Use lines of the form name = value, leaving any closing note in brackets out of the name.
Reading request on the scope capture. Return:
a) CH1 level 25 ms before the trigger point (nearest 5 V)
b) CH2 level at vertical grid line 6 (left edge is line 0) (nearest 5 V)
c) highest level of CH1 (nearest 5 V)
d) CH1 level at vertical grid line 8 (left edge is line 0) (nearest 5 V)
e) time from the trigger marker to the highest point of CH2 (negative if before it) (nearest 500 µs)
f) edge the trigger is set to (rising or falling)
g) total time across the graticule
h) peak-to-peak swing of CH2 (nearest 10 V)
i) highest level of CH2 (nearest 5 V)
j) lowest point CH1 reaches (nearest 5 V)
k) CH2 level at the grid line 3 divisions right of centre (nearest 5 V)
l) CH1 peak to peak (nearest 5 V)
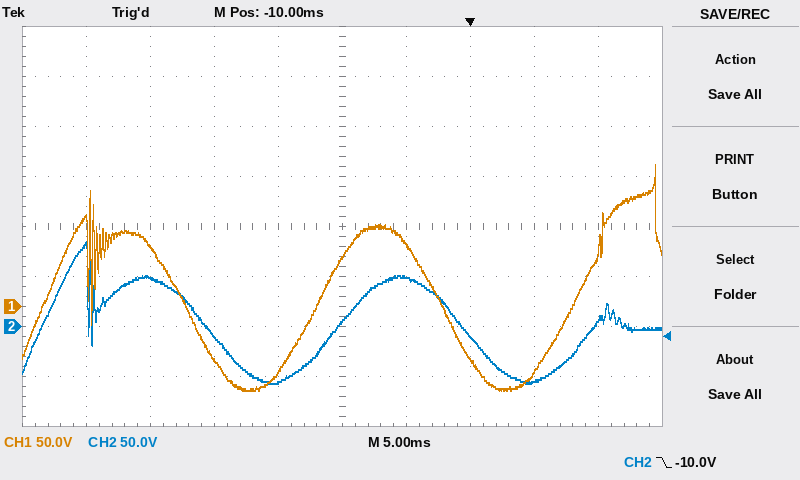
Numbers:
CH1 level 25 ms before the trigger point = 60 V
CH2 level at vertical grid line 6 (left edge is line 0) = 50 V
highest level of CH1 = 140 V
CH1 level at vertical grid line 8 (left edge is line 0) = -65 V
time from the trigger marker to the highest point of CH2 (negative if before it) = -30.0 ms
edge the trigger is set to = falling
total time across the graticule = 50 ms
peak-to-peak swing of CH2 = 140 V
highest level of CH2 = 85 V
lowest point CH1 reaches = -85 V
CH2 level at the grid line 3 divisions right of centre = -55 V
CH1 peak to peak = 225 V
